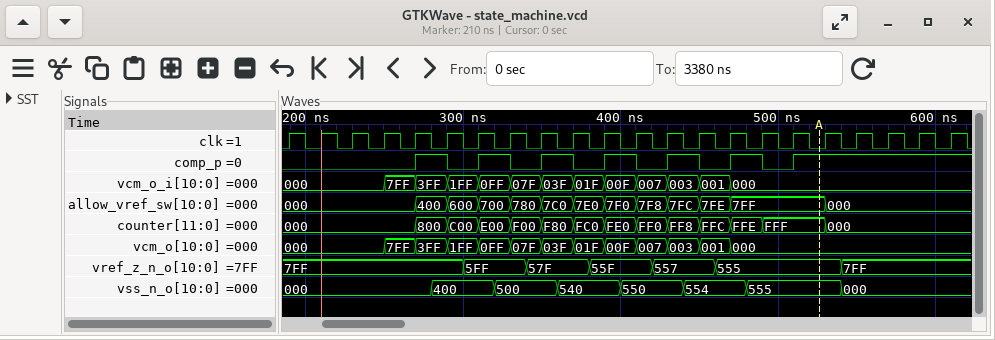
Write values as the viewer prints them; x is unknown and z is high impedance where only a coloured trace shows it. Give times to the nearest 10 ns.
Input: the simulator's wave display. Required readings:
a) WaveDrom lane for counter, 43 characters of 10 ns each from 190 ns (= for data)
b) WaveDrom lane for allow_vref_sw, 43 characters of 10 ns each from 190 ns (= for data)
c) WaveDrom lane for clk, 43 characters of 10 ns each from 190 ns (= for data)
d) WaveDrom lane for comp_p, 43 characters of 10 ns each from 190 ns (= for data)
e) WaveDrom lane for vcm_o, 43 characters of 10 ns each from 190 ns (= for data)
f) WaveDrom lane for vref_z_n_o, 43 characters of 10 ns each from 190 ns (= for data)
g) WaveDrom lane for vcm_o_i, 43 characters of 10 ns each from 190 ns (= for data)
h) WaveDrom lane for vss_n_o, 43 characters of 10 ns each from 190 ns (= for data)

{name: 'counter', wave: '=.......=.=.=.=.=.=.=.=.=.=.=.=...=........', data: '000 800 C00 E00 F00 F80 FC0 FE0 FF0 FF8 FFC FFE FFF 000'}
{name: 'allow_vref_sw', wave: '=.......=.=.=.=.=.=.=.=.=.=.=.....=........', data: '000 400 600 700 780 7C0 7E0 7F0 7F8 7FC 7FE 7FF 000'}
{name: 'clk', wave: '1010101010101010101010101010101010101010101'}
{name: 'comp_p', wave: '0.......1.0.1.0.1.0.1.0.1.0.1.0.1..........'}
{name: 'vcm_o', wave: '=.....=.=.=.=.=.=.=.=.=.=.=.=..............', data: '000 7FF 3FF 1FF 0FF 07F 03F 01F 00F 007 003 001 000'}
{name: 'vref_z_n_o', wave: '=..........=...=...=...=...=.......=.......', data: '7FF 5FF 57F 55F 557 555 7FF'}
{name: 'vcm_o_i', wave: '=.....=.=.=.=.=.=.=.=.=.=.=.=..............', data: '000 7FF 3FF 1FF 0FF 07F 03F 01F 00F 007 003 001 000'}
{name: 'vss_n_o', wave: '=........=...=...=...=...=...=.....=.......', data: '000 400 500 540 550 554 555 000'}
